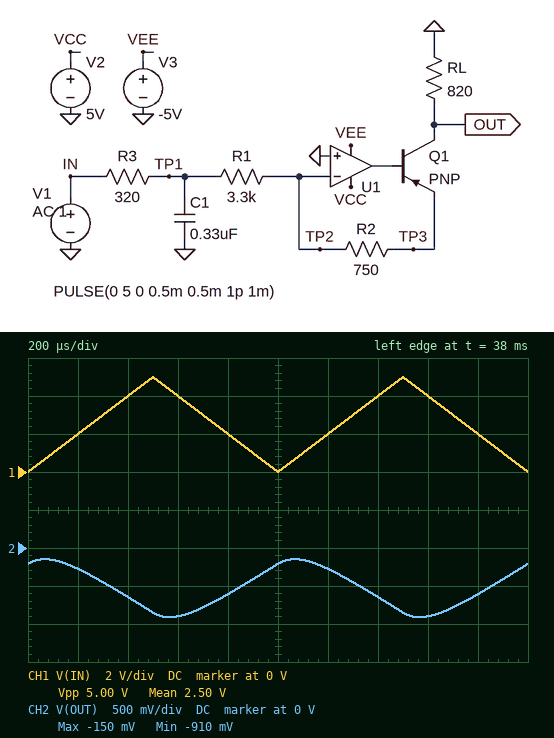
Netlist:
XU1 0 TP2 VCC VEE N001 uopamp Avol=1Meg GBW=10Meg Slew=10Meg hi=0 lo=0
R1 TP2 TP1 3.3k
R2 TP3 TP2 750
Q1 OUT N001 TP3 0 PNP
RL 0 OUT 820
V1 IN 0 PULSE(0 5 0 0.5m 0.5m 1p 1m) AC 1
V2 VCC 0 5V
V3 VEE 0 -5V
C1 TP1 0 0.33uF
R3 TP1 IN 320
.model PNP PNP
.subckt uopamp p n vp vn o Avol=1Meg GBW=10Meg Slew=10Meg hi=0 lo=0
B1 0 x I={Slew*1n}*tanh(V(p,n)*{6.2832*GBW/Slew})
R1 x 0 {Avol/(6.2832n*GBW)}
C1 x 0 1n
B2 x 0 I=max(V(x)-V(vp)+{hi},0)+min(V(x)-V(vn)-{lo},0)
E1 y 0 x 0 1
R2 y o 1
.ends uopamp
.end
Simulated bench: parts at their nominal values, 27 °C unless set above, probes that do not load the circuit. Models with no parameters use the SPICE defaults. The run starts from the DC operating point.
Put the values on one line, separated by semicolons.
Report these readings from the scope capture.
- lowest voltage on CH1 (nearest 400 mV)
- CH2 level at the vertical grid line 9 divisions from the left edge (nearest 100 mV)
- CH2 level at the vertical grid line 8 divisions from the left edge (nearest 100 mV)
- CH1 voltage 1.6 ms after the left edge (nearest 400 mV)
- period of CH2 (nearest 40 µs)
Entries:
0 V; -600 mV; -900 mV; 4.0 V; 1.00 ms
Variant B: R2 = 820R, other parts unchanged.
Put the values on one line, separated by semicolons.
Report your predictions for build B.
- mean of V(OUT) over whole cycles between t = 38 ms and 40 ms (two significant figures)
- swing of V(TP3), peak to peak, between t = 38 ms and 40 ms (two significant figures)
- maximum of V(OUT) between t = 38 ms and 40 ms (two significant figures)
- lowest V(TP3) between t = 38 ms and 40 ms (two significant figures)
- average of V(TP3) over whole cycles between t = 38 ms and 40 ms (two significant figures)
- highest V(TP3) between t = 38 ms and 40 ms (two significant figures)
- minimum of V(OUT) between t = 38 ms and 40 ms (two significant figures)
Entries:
-580 mV; 830 mV; -160 mV; -980 mV; -570 mV; -150 mV; -990 mV
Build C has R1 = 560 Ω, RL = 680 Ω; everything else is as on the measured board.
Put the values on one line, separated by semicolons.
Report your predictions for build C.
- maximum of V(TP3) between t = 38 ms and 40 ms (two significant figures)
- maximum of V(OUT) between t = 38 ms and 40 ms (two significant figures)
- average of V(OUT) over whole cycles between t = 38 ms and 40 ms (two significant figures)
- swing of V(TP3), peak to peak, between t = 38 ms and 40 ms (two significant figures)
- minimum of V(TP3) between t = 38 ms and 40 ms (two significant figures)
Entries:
-400 mV; -410 mV; -2.1 V; 3.5 V; -3.9 V
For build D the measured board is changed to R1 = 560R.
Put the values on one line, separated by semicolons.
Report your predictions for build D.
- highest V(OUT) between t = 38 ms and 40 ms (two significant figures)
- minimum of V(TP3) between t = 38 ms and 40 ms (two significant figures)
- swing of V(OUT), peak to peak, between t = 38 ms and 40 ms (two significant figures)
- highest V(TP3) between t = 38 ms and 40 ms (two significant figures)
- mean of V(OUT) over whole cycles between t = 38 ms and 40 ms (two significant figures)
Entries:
-410 mV; -3.9 V; 3.5 V; -400 mV; -2.1 V
